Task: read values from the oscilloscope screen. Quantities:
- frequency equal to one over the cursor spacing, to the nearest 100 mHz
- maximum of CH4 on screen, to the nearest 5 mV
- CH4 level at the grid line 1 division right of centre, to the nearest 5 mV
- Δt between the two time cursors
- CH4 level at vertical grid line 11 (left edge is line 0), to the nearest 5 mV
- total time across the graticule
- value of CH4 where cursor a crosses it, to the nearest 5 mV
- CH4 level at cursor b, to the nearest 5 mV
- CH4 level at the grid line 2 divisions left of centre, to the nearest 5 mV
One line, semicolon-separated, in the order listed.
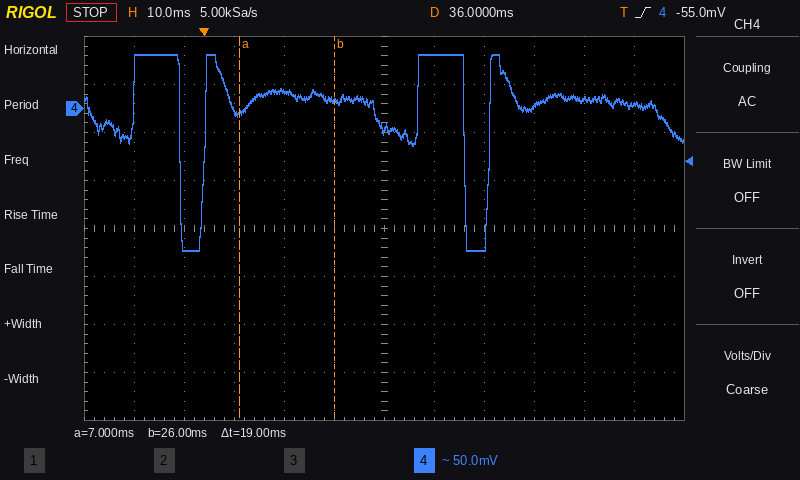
52.6 Hz; 55 mV; 55 mV; 19 ms; 5 mV; 120 ms; -5 mV; 10 mV; 20 mV
